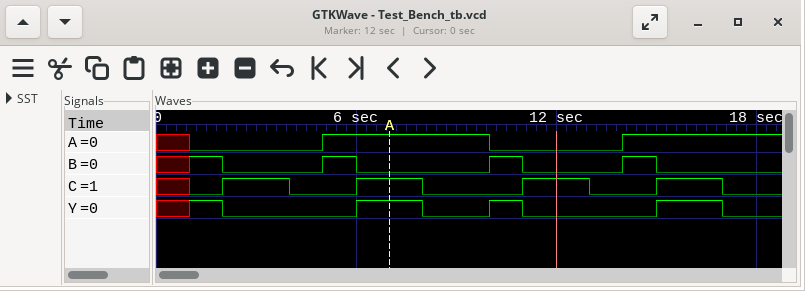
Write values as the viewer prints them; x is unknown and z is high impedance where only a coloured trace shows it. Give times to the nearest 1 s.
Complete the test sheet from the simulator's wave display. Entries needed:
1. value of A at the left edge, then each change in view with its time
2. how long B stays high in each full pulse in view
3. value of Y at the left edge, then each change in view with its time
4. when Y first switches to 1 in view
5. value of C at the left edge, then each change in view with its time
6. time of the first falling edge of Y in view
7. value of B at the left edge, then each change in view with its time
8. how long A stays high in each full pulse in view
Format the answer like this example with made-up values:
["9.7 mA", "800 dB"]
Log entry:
["x, 0 at 1 s, 1 at 5 s, 0 at 10 s, 1 at 14 s", "1 s, 1 s, 1 s", "x, 1 at 1 s, 0 at 2 s, 1 at 6 s, 0 at 8 s, 1 at 10 s, 0 at 11 s, 1 at 15 s, 0 at 17 s", "1 s", "x, 0 at 1 s, 1 at 2 s, 0 at 4 s, 1 at 6 s, 0 at 8 s, 1 at 11 s, 0 at 13 s, 1 at 15 s, 0 at 17 s", "2 s", "x, 1 at 1 s, 0 at 2 s, 1 at 5 s, 0 at 6 s, 1 at 10 s, 0 at 11 s, 1 at 14 s, 0 at 15 s", "5 s"]
